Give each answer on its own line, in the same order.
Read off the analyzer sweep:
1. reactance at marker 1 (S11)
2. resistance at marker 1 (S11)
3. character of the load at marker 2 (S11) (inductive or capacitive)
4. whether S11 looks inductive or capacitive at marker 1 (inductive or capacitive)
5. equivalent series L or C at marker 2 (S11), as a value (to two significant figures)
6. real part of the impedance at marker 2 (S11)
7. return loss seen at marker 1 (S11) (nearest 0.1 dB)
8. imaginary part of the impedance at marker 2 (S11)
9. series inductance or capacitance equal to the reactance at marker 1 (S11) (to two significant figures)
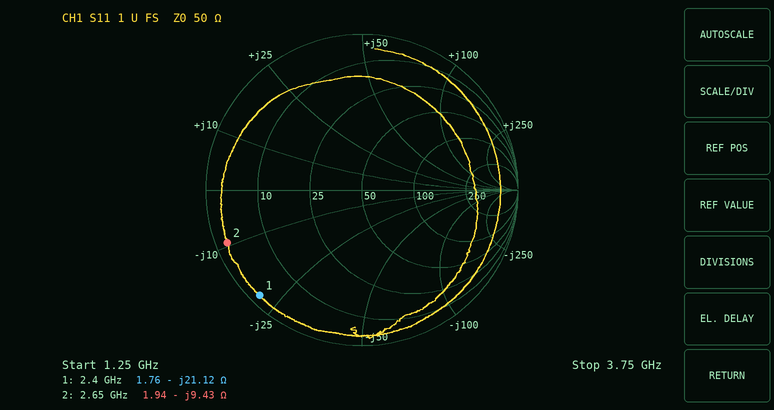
-21.12 Ω
1.76 Ω
capacitive
capacitive
6.4 pF
1.94 Ω
0.5 dB
-9.43 Ω
3.1 pF
